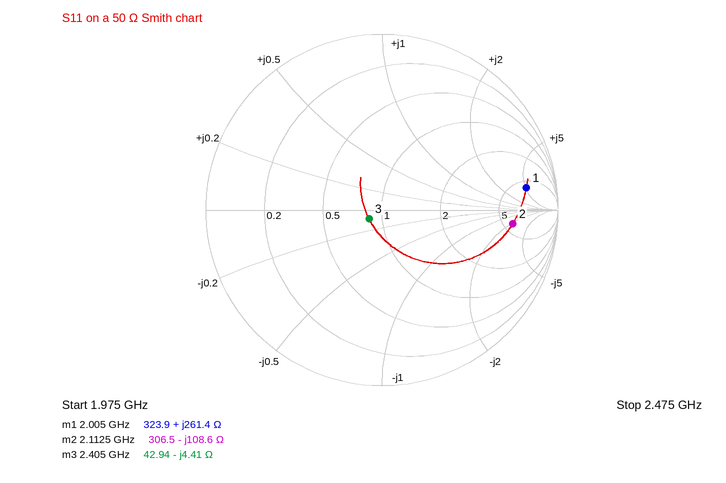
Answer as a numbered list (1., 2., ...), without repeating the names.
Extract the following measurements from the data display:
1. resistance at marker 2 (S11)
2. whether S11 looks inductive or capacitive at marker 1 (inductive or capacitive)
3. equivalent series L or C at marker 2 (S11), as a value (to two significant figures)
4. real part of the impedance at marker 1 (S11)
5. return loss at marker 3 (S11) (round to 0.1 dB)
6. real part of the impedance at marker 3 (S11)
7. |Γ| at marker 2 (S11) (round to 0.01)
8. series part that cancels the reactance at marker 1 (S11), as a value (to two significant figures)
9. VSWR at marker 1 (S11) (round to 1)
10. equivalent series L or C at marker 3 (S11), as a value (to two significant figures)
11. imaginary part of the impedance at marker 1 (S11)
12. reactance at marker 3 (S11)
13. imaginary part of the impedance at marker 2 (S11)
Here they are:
1. 306.5 Ω
2. inductive
3. 690 fF
4. 323.9 Ω
5. 21.0 dB
6. 42.94 Ω
7. 0.75
8. 300 fF
9. 11
10. 15 pF
11. +261.4 Ω
12. -4.41 Ω
13. -108.6 Ω
